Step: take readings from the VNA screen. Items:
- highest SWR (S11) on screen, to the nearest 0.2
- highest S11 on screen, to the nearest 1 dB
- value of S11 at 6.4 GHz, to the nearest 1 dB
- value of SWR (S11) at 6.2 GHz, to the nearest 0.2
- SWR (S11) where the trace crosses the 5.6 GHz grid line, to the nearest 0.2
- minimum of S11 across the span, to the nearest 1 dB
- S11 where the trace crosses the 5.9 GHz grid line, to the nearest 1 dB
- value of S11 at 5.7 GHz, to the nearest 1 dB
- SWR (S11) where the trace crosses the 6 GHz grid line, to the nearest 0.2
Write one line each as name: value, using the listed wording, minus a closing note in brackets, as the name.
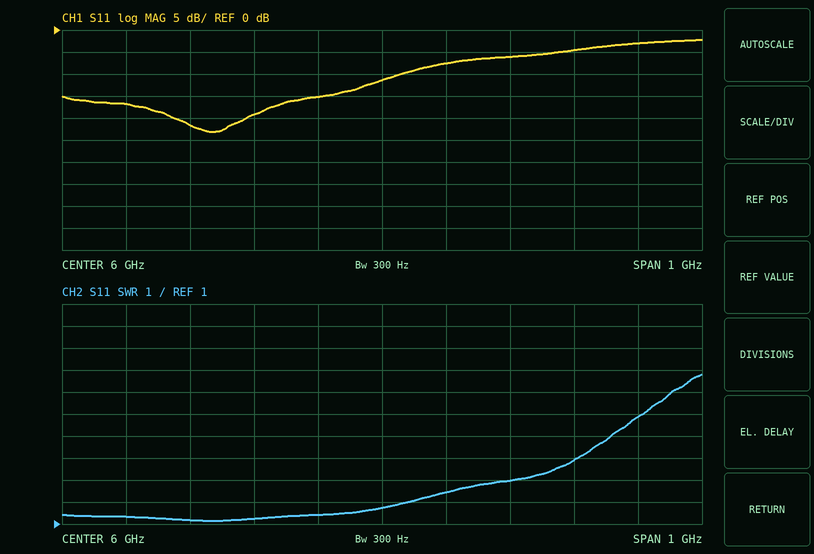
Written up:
highest SWR (S11) on screen, to the nearest 0.2: 7.8
highest S11 on screen, to the nearest 1 dB: -2 dB
value of S11 at 6.4 GHz, to the nearest 1 dB: -3 dB
value of SWR (S11) at 6.2 GHz, to the nearest 0.2: 3.0
SWR (S11) where the trace crosses the 5.6 GHz grid line, to the nearest 0.2: 1.4
minimum of S11 across the span, to the nearest 1 dB: -23 dB
S11 where the trace crosses the 5.9 GHz grid line, to the nearest 1 dB: -15 dB
value of S11 at 5.7 GHz, to the nearest 1 dB: -22 dB
SWR (S11) where the trace crosses the 6 GHz grid line, to the nearest 0.2: 1.8
